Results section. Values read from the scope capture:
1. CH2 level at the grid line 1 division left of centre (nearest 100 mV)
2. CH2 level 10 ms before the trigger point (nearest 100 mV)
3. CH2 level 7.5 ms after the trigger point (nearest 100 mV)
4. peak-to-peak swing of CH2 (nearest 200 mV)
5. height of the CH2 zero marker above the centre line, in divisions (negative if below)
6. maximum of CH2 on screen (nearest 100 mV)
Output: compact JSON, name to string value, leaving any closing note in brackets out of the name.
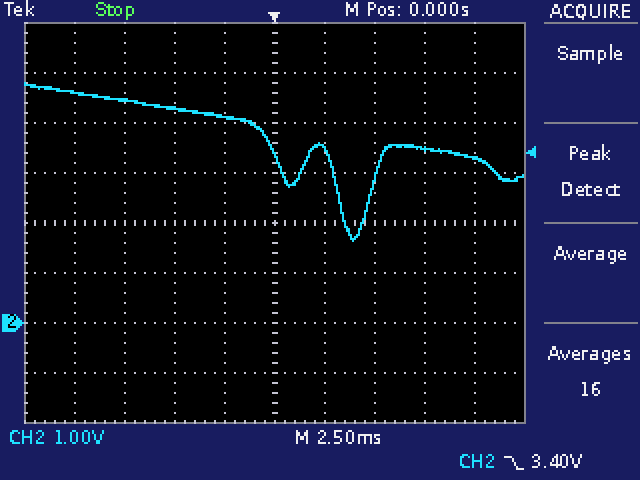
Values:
{"CH2 level at the grid line 1 division left of centre": "4.1 V", "CH2 level 10 ms before the trigger point": "4.6 V", "CH2 level 7.5 ms after the trigger point": "3.5 V", "peak-to-peak swing of CH2": "3.2 V", "height of the CH2 zero marker above the centre line, in divisions": "-2.0 div", "maximum of CH2 on screen": "4.8 V"}
